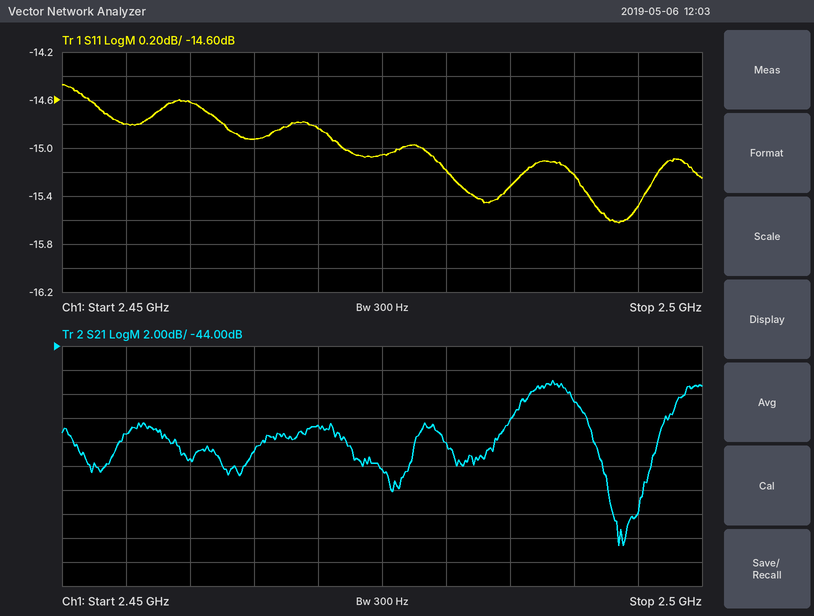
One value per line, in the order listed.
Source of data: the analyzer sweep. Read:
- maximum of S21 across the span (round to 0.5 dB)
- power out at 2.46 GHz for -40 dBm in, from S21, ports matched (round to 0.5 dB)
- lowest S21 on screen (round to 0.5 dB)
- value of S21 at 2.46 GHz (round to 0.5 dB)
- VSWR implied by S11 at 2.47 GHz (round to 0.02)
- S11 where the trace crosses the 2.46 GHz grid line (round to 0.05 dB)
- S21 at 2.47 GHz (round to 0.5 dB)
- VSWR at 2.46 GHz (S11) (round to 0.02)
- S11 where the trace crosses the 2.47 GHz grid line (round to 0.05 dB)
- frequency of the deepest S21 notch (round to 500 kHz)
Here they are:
-47.0 dB
-93.5 dBm
-60.5 dB
-53.5 dB
1.44
-14.60 dB
-50.5 dB
1.46
-14.85 dB
2.4935 GHz
